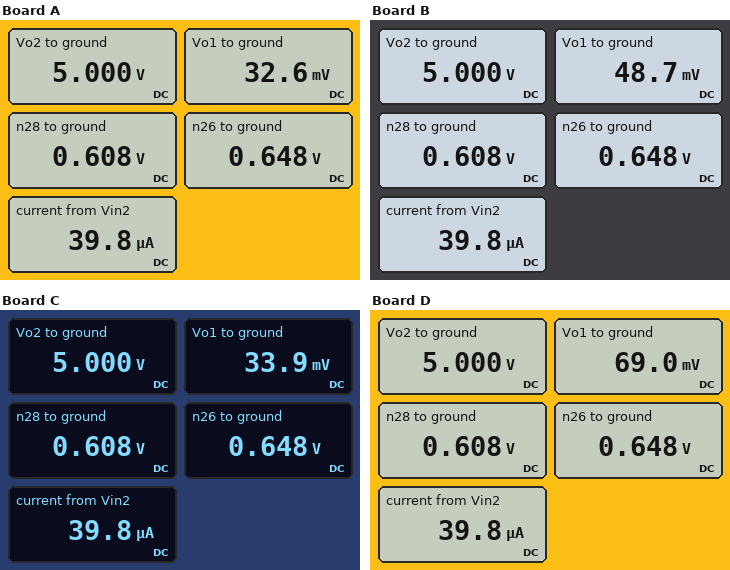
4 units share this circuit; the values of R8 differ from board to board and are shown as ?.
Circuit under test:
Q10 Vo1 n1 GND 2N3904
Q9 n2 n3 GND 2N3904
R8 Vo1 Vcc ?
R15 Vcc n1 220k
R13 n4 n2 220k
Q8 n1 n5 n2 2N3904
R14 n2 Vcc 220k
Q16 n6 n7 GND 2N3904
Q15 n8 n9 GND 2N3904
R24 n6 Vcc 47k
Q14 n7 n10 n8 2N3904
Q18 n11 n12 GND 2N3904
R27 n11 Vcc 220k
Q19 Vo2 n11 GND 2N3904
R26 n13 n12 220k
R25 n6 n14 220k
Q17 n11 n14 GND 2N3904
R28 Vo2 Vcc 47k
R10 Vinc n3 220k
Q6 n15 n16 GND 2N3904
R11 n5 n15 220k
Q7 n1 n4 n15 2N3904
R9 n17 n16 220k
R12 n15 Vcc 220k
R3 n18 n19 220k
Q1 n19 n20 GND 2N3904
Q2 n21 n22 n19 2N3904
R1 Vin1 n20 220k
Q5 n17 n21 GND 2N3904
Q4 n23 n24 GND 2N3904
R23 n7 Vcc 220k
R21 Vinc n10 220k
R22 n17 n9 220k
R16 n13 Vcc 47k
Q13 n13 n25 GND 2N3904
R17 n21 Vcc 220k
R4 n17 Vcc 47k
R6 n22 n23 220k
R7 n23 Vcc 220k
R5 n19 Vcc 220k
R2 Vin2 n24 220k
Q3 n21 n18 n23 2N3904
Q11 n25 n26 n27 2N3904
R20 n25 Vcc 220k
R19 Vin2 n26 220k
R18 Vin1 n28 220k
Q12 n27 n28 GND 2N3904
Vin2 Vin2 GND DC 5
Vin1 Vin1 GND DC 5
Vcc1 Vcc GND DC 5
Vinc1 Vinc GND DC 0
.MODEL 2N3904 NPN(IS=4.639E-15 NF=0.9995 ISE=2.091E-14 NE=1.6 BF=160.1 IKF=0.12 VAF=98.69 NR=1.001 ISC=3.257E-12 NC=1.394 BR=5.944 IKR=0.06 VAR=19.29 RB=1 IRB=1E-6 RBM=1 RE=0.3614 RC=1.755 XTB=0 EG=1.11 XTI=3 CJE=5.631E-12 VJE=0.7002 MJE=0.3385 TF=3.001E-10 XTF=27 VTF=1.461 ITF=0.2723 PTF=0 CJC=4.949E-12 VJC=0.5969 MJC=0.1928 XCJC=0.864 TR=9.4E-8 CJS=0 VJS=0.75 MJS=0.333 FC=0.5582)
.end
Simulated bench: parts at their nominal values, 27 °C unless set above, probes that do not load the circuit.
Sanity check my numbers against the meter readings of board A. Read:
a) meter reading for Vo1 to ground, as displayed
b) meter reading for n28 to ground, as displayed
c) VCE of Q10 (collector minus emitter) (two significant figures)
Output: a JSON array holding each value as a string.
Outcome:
["32.6 mV", "0.608 V", "33 mV"]
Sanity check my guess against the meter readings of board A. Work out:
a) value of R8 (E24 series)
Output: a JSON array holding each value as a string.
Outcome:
["150 kΩ"]
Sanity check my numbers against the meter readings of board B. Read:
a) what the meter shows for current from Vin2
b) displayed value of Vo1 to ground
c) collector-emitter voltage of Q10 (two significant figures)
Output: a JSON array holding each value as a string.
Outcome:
["39.8 µA", "48.7 mV", "49 mV"]
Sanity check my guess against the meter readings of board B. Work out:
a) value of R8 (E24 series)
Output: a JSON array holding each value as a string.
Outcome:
["43 kΩ"]
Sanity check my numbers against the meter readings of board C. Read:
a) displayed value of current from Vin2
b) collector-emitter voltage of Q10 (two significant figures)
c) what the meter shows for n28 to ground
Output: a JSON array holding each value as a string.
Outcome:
["39.8 µA", "34 mV", "0.608 V"]
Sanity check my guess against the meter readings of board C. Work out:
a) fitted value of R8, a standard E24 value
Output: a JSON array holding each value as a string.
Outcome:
["130 kΩ"]
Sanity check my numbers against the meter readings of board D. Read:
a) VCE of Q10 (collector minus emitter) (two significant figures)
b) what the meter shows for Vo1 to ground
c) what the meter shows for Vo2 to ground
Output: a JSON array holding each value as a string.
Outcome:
["69 mV", "69.0 mV", "5.000 V"]
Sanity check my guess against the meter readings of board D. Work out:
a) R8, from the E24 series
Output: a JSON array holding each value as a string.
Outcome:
["16 kΩ"]
